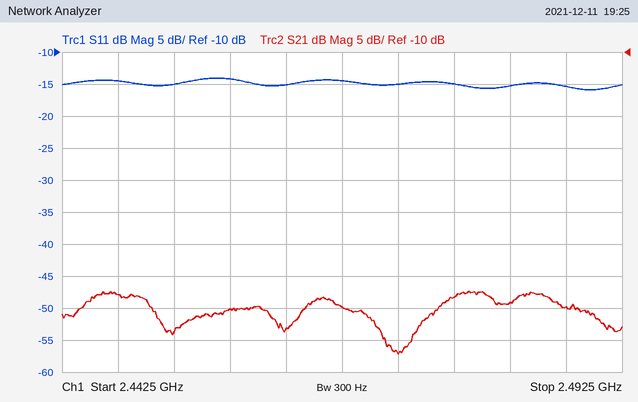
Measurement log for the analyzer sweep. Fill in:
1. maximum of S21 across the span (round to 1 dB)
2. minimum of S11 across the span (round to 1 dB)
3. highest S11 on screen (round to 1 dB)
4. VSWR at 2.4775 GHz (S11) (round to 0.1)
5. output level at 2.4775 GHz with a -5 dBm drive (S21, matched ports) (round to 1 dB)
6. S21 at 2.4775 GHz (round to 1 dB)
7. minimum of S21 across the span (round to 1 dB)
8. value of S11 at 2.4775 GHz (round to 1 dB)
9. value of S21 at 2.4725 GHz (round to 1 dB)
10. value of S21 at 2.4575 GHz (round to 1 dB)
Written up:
-47 dB
-16 dB
-14 dB
1.4
-53 dBm
-48 dB
-57 dB
-15 dB
-57 dB
-50 dB
